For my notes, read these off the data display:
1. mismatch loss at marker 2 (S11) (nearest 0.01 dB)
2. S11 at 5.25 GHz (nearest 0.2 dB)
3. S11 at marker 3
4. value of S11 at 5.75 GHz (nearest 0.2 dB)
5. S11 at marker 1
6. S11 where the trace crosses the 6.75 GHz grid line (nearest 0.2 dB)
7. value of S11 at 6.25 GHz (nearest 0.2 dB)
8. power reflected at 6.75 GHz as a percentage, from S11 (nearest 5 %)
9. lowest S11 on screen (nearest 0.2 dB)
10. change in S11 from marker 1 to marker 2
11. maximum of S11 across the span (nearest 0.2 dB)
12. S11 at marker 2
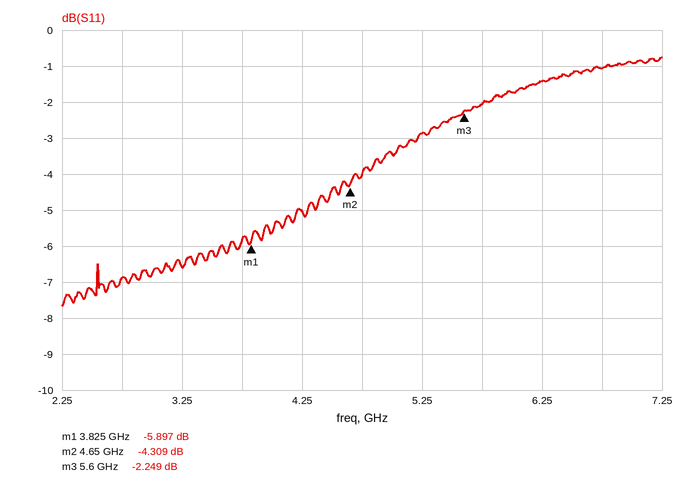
2.01 dB
-2.8 dB
-2.249 dB
-2.0 dB
-5.897 dB
-1.0 dB
-1.4 dB
80 %
-7.6 dB
1.588 dB
-0.8 dB
-4.309 dB
